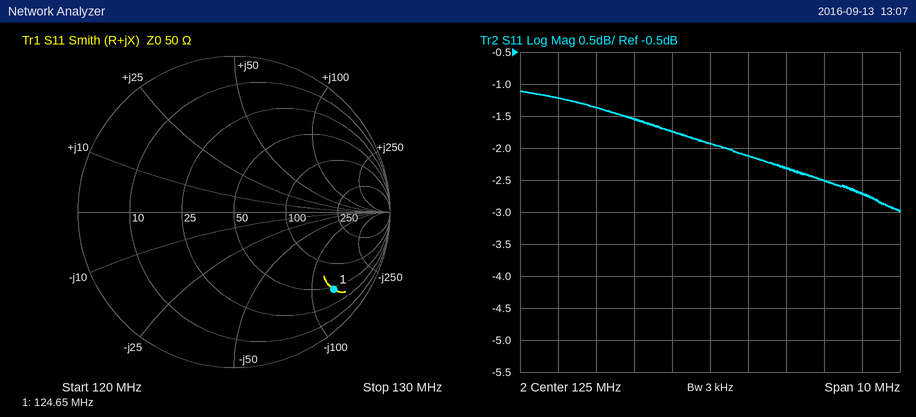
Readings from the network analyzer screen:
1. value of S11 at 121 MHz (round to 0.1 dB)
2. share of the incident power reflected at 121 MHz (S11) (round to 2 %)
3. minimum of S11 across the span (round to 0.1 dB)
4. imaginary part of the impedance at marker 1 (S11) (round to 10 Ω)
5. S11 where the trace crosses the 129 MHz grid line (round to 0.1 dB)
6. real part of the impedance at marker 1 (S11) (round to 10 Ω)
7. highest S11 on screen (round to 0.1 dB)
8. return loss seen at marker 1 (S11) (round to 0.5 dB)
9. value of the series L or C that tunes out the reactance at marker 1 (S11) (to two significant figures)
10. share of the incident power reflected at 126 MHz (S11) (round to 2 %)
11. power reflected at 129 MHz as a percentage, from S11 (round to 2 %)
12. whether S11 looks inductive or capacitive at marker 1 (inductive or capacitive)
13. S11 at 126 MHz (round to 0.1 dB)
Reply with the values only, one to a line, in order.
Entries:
-1.2 dB
76 %
-3.0 dB
-130 Ω
-2.7 dB
50 Ω
-1.1 dB
2.0 dB
170 nH
62 %
54 %
capacitive
-2.1 dB
